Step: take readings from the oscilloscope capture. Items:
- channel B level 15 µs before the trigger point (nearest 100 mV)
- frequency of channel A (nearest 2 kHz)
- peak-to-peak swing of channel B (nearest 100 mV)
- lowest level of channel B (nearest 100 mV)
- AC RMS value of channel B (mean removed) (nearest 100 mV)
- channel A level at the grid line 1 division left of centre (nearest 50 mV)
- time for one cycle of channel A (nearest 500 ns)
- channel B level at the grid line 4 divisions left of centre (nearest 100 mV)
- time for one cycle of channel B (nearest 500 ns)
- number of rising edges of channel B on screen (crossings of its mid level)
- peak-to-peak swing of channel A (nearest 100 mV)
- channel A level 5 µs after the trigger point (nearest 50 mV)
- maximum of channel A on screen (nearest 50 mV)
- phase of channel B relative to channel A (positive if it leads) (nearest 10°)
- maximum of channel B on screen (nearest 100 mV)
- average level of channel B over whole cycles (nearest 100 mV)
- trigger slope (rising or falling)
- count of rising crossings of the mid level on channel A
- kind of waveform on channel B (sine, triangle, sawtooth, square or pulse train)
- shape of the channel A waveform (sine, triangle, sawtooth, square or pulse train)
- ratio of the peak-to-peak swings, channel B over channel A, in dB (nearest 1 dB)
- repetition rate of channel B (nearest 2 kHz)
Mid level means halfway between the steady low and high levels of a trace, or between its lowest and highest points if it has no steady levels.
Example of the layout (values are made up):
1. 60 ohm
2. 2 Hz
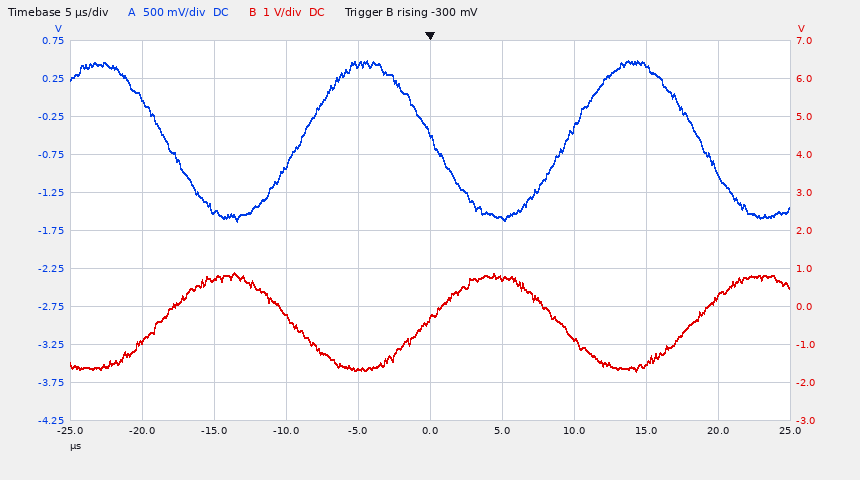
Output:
1. 700 mV
2. 54 kHz
3. 2.6 V
4. -1.7 V
5. 900 mV
6. 450 mV
7. 18.5 µs
8. -900 mV
9. 18.5 µs
10. 3
11. 2.10 V
12. -1.60 V
13. 500 mV
14. -170°
15. 900 mV
16. -400 mV
17. rising
18. 2
19. sine
20. sine
21. 2 dB
22. 54 kHz
